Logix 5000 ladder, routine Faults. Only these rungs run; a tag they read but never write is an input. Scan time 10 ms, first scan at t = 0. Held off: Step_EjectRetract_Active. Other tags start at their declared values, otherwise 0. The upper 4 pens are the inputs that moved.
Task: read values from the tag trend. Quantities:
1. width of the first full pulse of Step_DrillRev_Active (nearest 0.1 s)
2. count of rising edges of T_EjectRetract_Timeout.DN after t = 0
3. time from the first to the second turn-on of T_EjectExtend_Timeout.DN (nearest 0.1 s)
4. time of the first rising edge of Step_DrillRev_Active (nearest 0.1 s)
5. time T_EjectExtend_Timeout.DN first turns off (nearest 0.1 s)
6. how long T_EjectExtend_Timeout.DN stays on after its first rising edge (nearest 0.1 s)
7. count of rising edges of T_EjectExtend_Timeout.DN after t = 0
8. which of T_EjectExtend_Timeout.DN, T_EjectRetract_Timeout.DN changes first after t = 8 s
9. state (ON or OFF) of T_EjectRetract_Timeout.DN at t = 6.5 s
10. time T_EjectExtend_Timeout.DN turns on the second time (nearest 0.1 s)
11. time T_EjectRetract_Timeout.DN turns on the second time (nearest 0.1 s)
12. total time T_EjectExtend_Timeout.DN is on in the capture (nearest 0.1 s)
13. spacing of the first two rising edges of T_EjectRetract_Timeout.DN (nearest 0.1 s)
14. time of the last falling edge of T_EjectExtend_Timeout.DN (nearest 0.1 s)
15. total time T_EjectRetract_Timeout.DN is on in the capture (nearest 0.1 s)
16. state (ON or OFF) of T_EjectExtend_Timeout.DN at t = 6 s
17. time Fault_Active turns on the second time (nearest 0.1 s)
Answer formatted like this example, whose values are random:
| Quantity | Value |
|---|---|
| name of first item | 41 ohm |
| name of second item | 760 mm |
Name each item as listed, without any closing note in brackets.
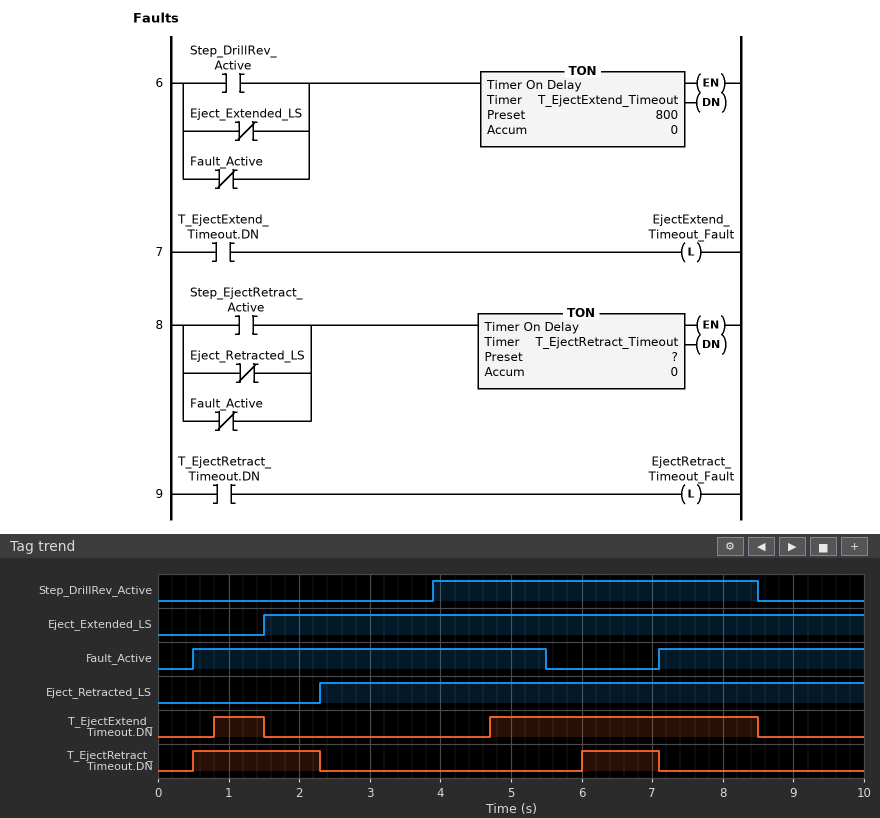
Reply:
| Quantity | Value |
|---|---|
| width of the first full pulse of Step_DrillRev_Active | 4.6 s |
| count of rising edges of T_EjectRetract_Timeout.DN after t = 0 | 2 |
| time from the first to the second turn-on of T_EjectExtend_Timeout.DN | 3.9 s |
| time of the first rising edge of Step_DrillRev_Active | 3.9 s |
| time T_EjectExtend_Timeout.DN first turns off | 1.5 s |
| how long T_EjectExtend_Timeout.DN stays on after its first rising edge | 0.7 s |
| count of rising edges of T_EjectExtend_Timeout.DN after t = 0 | 2 |
| which of T_EjectExtend_Timeout.DN, T_EjectRetract_Timeout.DN changes first after t = 8 s | T_EjectExtend_Timeout.DN |
| state (ON or OFF) of T_EjectRetract_Timeout.DN at t = 6.5 s | ON |
| time T_EjectExtend_Timeout.DN turns on the second time | 4.7 s |
| time T_EjectRetract_Timeout.DN turns on the second time | 6.0 s |
| total time T_EjectExtend_Timeout.DN is on in the capture | 4.5 s |
| spacing of the first two rising edges of T_EjectRetract_Timeout.DN | 5.5 s |
| time of the last falling edge of T_EjectExtend_Timeout.DN | 8.5 s |
| total time T_EjectRetract_Timeout.DN is on in the capture | 2.9 s |
| state (ON or OFF) of T_EjectExtend_Timeout.DN at t = 6 s | ON |
| time Fault_Active turns on the second time | 7.1 s |
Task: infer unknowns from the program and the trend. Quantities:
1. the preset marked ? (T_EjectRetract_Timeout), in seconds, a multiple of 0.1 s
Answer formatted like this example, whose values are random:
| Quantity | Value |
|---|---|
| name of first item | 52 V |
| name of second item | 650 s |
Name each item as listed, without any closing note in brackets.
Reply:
| Quantity | Value |
|---|---|
| the preset marked ? (T_EjectRetract_Timeout), in seconds, a multiple of 0.1 s | 0.5 s |
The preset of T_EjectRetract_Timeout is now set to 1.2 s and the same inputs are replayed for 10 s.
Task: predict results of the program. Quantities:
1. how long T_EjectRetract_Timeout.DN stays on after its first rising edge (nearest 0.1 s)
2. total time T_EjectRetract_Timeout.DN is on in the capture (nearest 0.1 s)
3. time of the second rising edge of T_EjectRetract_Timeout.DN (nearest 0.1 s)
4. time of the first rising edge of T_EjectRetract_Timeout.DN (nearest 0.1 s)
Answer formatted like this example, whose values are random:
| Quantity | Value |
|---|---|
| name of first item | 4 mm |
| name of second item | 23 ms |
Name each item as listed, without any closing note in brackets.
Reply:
| Quantity | Value |
|---|---|
| how long T_EjectRetract_Timeout.DN stays on after its first rising edge | 1.1 s |
| total time T_EjectRetract_Timeout.DN is on in the capture | 1.5 s |
| time of the second rising edge of T_EjectRetract_Timeout.DN | 6.7 s |
| time of the first rising edge of T_EjectRetract_Timeout.DN | 1.2 s |
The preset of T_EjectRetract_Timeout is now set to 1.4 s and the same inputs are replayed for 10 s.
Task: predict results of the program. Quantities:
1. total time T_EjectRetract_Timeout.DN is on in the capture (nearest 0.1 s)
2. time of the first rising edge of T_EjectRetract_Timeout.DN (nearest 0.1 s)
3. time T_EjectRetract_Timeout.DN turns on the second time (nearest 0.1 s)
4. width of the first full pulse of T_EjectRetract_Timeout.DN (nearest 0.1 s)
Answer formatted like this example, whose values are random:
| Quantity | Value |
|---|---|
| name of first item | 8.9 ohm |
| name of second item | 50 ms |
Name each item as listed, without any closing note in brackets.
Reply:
| Quantity | Value |
|---|---|
| total time T_EjectRetract_Timeout.DN is on in the capture | 1.1 s |
| time of the first rising edge of T_EjectRetract_Timeout.DN | 1.4 s |
| time T_EjectRetract_Timeout.DN turns on the second time | 6.9 s |
| width of the first full pulse of T_EjectRetract_Timeout.DN | 0.9 s |
